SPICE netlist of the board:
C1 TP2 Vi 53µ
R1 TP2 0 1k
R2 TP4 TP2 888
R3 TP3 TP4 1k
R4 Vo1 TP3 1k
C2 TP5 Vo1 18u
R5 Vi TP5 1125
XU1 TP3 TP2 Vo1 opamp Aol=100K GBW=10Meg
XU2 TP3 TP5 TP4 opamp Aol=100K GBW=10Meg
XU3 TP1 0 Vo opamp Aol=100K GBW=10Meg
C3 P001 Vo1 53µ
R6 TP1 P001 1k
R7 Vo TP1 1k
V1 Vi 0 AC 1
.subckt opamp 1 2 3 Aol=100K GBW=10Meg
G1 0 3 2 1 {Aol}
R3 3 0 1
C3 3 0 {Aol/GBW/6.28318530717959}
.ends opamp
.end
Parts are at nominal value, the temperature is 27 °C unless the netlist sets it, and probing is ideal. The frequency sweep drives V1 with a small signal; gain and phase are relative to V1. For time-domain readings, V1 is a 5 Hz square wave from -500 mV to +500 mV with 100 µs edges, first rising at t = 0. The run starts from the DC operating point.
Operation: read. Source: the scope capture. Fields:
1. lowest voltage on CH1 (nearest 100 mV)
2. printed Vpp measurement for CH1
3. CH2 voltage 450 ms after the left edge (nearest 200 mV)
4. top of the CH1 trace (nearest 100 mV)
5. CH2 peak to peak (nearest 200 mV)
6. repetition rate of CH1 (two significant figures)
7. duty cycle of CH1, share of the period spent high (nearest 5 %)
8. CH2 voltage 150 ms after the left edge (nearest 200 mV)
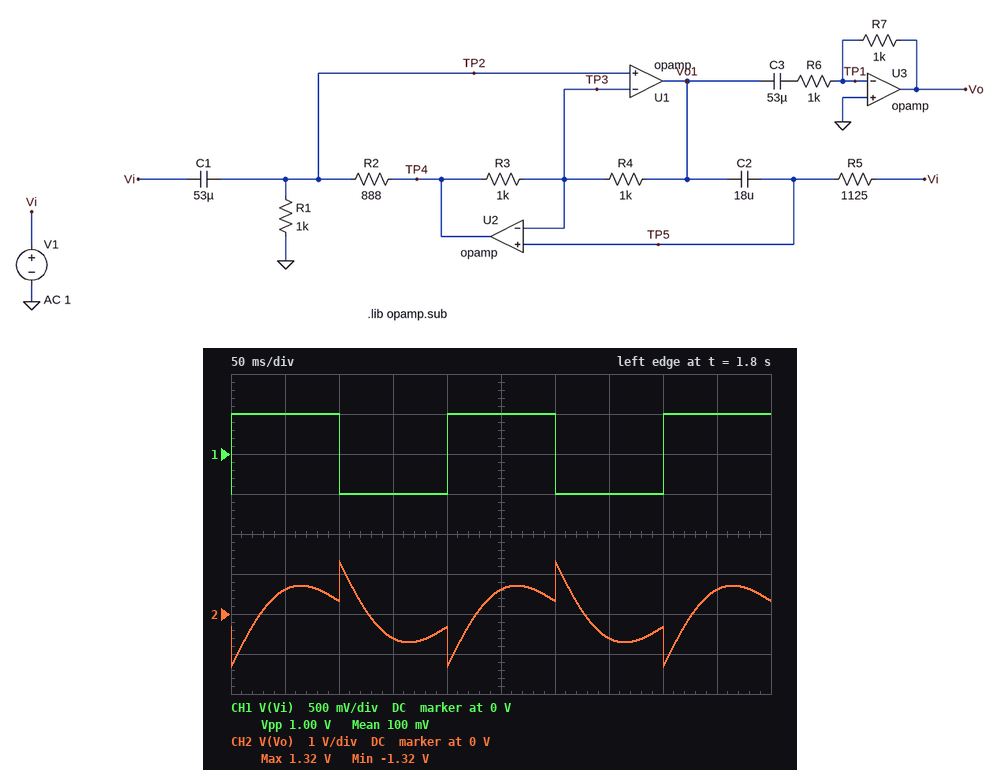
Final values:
-500 mV
1.00 V
600 mV
500 mV
2.6 V
5.0 Hz
50 %
-600 mV
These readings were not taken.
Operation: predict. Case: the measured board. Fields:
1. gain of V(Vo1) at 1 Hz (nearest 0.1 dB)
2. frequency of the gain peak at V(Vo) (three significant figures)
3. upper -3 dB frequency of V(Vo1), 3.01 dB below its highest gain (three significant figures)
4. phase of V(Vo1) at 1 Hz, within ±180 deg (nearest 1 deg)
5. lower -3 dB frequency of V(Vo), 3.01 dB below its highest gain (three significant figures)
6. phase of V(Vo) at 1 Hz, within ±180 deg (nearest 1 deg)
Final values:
-22.3 dB
5.96 Hz
11.8 Hz
-7 deg
4.60 Hz
-115 deg
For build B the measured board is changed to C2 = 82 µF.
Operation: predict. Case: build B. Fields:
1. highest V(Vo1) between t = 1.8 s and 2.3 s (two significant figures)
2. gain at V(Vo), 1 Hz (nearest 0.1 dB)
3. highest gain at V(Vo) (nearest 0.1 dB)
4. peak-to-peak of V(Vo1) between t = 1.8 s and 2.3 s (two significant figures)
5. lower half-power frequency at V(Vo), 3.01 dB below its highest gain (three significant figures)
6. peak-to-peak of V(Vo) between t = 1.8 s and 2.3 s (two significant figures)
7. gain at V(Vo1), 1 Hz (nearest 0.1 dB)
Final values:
980 mV
-34.3 dB
0 dB
2.0 V
3.45 Hz
2.4 V
-24.3 dB
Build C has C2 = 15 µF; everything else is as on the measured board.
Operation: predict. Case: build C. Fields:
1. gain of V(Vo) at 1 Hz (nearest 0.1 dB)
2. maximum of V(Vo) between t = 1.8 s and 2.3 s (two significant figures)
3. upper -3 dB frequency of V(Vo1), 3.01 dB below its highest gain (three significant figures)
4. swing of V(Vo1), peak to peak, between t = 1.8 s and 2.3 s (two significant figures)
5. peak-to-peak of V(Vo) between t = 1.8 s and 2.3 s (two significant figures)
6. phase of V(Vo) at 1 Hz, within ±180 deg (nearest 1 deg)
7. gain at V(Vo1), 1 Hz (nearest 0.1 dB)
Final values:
-31.6 dB
1.1 V
10.7 Hz
2.7 V
2.2 V
-114 deg
-21.6 dB
